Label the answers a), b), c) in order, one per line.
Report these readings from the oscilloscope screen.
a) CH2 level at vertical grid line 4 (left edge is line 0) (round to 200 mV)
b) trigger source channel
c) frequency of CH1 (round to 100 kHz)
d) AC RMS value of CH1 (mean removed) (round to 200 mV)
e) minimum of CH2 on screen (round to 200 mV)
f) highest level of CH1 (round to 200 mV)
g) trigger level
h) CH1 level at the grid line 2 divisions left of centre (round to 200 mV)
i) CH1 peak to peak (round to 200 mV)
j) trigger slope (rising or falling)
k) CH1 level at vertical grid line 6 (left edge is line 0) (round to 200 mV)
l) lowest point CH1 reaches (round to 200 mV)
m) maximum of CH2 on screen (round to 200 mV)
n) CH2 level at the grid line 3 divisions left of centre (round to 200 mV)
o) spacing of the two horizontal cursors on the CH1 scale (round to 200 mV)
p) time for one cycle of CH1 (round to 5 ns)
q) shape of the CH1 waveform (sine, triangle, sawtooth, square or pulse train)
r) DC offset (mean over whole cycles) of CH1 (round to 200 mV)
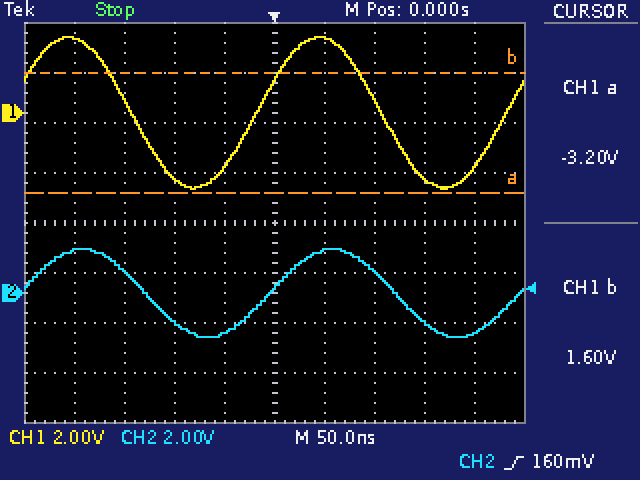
a) -1.6 V
b) CH2
c) 4.0 MHz
d) 2.2 V
e) -1.8 V
f) 3.0 V
g) 160 mV
h) -2.6 V
i) 6.0 V
j) rising
k) 3.0 V
l) -3.0 V
m) 1.8 V
n) 800 mV
o) 4.8 V
p) 250 ns
q) sine
r) 0.0 V
